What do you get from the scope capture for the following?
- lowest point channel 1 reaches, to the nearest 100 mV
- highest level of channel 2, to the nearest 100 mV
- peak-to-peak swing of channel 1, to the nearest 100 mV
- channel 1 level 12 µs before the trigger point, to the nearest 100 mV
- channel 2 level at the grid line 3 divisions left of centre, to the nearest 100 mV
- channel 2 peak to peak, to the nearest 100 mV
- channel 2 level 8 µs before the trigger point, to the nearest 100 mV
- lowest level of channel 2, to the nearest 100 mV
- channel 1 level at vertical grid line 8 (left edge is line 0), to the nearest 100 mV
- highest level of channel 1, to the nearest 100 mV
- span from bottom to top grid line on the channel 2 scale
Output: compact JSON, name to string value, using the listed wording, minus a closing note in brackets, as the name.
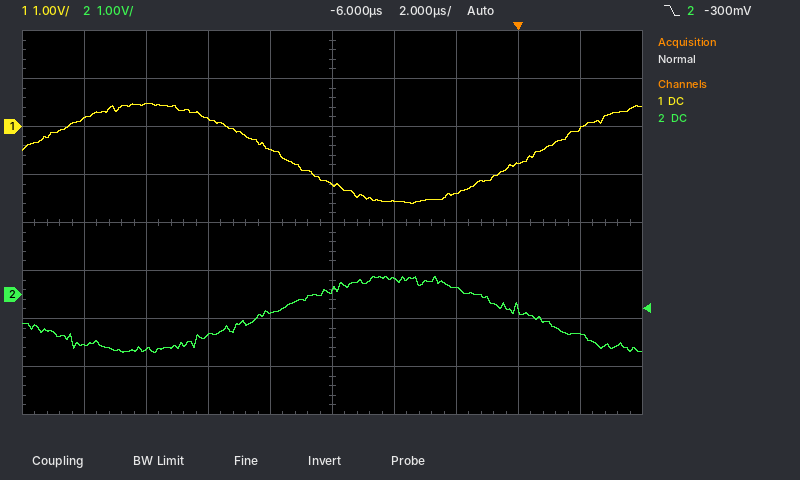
{"lowest point channel 1 reaches, to the nearest 100 mV": "-1.6 V", "highest level of channel 2, to the nearest 100 mV": "400 mV", "peak-to-peak swing of channel 1, to the nearest 100 mV": "2.1 V", "channel 1 level 12 µs before the trigger point, to the nearest 100 mV": "500 mV", "channel 2 level at the grid line 3 divisions left of centre, to the nearest 100 mV": "-1.1 V", "channel 2 peak to peak, to the nearest 100 mV": "1.6 V", "channel 2 level 8 µs before the trigger point, to the nearest 100 mV": "-400 mV", "lowest level of channel 2, to the nearest 100 mV": "-1.2 V", "channel 1 level at vertical grid line 8 (left edge is line 0), to the nearest 100 mV": "-800 mV", "highest level of channel 1, to the nearest 100 mV": "500 mV", "span from bottom to top grid line on the channel 2 scale": "8 V"}
